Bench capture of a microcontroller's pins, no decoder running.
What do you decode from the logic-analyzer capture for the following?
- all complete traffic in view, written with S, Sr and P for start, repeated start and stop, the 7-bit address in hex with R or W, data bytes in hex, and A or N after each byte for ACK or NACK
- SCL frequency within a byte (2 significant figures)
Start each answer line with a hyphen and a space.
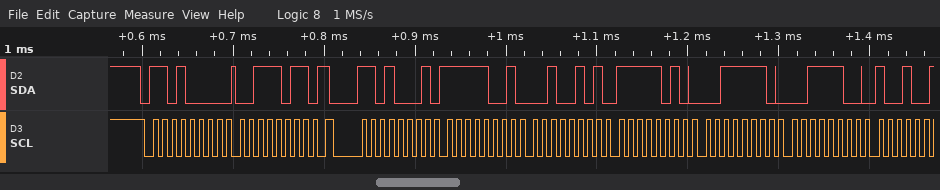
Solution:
- S 68W A 3B A Sr 68R A F9 A 25 A FA A 3E A 3C A
- 100 kHz
